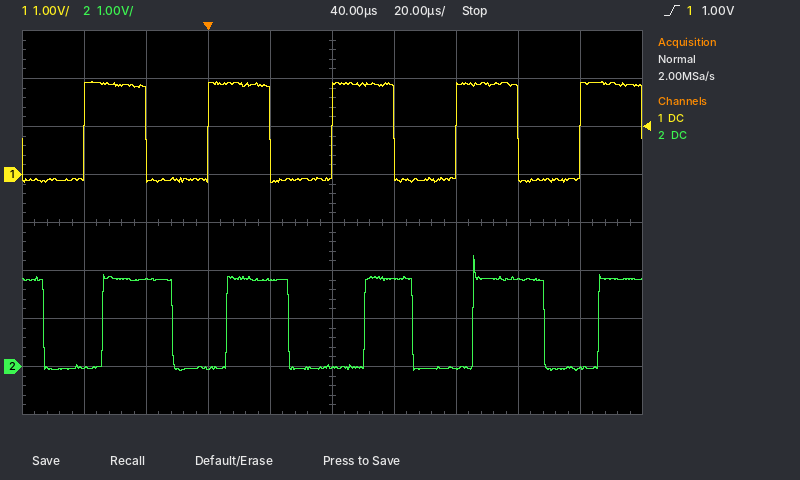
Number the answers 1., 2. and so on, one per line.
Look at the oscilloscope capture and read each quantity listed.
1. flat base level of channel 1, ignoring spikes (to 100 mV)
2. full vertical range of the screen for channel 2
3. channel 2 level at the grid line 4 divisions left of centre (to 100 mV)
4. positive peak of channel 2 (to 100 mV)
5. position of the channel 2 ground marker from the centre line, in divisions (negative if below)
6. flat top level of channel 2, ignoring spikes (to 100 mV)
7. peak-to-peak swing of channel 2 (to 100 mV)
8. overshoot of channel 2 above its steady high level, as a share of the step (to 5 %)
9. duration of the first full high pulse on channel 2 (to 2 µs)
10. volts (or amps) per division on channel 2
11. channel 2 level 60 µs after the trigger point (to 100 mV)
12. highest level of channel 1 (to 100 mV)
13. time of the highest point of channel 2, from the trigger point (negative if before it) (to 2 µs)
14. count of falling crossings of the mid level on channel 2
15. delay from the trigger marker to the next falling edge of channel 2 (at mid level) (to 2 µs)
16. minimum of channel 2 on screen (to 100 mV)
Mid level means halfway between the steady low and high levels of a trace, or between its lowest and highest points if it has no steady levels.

1. -100 mV
2. 8 V
3. 0.0 V
4. 2.3 V
5. -3.0 div
6. 1.8 V
7. 2.4 V
8. 25 %
9. 22 µs
10. 1 V
11. 1.8 V
12. 1.9 V
13. +86 µs
14. 5
15. 26 µs
16. -100 mV
